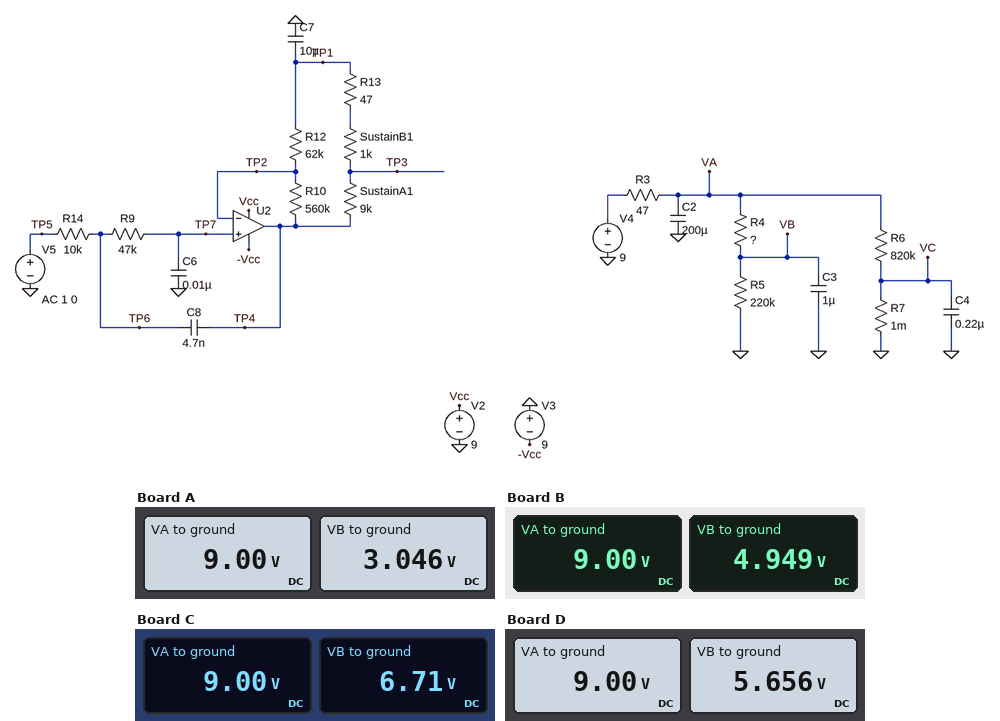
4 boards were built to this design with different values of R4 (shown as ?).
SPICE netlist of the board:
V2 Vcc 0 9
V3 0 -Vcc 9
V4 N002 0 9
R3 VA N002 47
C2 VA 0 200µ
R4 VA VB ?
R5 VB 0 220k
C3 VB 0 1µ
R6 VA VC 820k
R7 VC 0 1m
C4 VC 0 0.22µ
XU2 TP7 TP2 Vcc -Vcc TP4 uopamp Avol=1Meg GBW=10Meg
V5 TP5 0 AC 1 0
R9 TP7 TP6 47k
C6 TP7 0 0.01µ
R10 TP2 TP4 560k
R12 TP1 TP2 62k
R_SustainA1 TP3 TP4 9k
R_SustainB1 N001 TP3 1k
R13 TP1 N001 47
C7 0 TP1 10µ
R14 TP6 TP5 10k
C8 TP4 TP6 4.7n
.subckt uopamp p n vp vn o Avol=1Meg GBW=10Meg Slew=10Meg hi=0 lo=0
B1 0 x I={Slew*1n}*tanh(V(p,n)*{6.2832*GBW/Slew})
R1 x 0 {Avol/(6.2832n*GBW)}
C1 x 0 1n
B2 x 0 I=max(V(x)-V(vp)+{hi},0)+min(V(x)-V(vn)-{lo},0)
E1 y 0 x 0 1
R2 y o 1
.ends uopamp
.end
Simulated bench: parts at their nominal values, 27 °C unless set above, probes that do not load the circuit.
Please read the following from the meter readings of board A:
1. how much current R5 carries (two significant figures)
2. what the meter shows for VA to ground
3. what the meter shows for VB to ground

14 µA
9.00 V
3.046 V
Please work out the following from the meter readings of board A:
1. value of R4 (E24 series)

430 kΩ
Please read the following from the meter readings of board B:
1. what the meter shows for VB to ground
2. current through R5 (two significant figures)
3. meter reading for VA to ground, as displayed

4.949 V
22 µA
9.00 V
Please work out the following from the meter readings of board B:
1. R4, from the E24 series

180 kΩ
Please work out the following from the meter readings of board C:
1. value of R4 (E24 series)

75 kΩ
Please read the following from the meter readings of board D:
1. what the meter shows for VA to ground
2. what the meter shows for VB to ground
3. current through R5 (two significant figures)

9.00 V
5.656 V
26 µA
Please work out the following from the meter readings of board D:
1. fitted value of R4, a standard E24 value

130 kΩ
